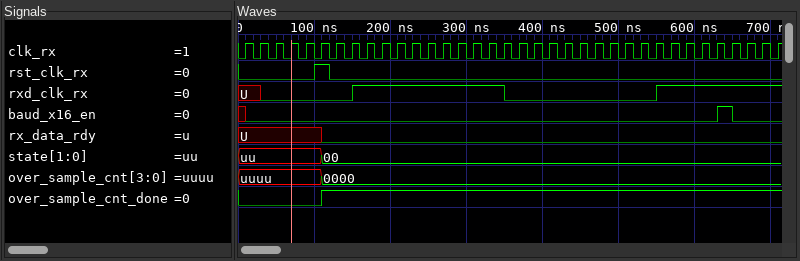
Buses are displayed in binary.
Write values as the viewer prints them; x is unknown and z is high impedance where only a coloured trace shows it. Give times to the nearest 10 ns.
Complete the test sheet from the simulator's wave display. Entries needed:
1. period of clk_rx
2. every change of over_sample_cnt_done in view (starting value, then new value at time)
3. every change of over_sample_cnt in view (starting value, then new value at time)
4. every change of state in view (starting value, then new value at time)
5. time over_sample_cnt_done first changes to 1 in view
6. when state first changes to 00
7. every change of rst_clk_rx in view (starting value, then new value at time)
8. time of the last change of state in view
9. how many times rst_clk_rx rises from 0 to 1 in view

20 ns
0, 1 at 110 ns
uuuu, 0000 at 110 ns
uu, 00 at 110 ns
110 ns
110 ns
0, 1 at 100 ns, 0 at 120 ns
110 ns
1
